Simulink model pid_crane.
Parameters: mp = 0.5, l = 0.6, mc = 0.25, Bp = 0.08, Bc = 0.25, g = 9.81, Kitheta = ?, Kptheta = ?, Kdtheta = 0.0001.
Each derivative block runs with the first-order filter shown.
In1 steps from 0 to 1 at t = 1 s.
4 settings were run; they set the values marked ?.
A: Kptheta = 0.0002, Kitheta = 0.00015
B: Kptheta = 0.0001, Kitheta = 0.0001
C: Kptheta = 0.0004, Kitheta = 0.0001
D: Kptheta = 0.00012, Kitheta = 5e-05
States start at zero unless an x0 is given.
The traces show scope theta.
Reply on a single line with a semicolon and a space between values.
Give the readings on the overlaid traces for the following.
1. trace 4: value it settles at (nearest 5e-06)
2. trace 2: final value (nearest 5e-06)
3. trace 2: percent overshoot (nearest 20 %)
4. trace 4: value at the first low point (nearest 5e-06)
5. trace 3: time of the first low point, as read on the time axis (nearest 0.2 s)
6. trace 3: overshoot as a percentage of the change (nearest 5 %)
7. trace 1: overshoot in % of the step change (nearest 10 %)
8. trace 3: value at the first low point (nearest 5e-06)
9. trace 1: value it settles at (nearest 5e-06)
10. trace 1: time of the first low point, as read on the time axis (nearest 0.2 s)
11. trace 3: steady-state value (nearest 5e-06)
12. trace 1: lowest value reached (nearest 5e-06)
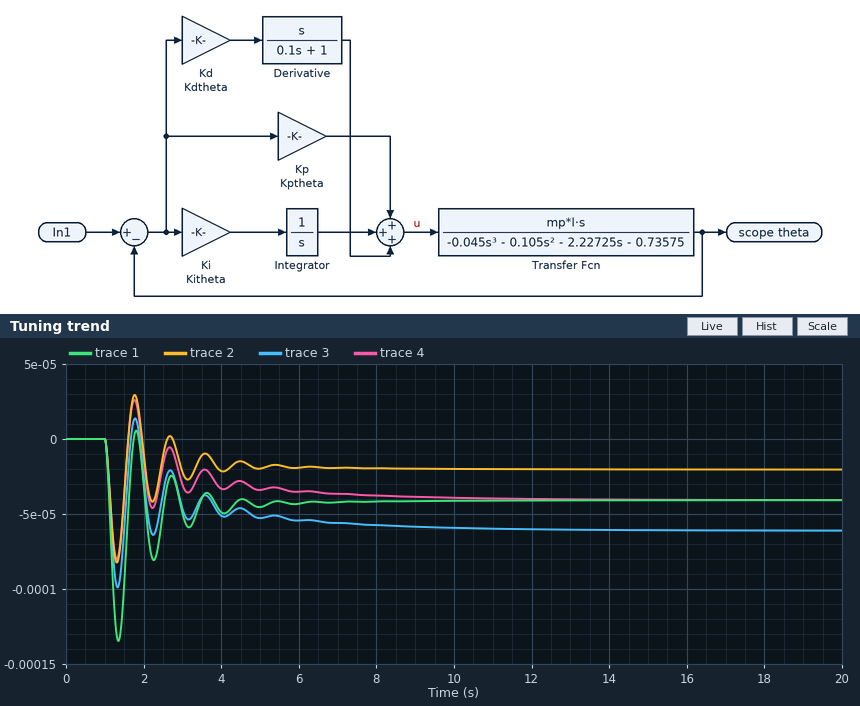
-0.000040; -0.000020; 300 %; -0.000080; 1.4 s; 60 %; 230 %; -0.000100; -0.000040; 1.4 s; -0.000060; -0.000135
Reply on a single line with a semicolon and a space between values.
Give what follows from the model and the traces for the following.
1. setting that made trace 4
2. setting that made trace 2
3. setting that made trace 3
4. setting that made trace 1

B; D; A; C
